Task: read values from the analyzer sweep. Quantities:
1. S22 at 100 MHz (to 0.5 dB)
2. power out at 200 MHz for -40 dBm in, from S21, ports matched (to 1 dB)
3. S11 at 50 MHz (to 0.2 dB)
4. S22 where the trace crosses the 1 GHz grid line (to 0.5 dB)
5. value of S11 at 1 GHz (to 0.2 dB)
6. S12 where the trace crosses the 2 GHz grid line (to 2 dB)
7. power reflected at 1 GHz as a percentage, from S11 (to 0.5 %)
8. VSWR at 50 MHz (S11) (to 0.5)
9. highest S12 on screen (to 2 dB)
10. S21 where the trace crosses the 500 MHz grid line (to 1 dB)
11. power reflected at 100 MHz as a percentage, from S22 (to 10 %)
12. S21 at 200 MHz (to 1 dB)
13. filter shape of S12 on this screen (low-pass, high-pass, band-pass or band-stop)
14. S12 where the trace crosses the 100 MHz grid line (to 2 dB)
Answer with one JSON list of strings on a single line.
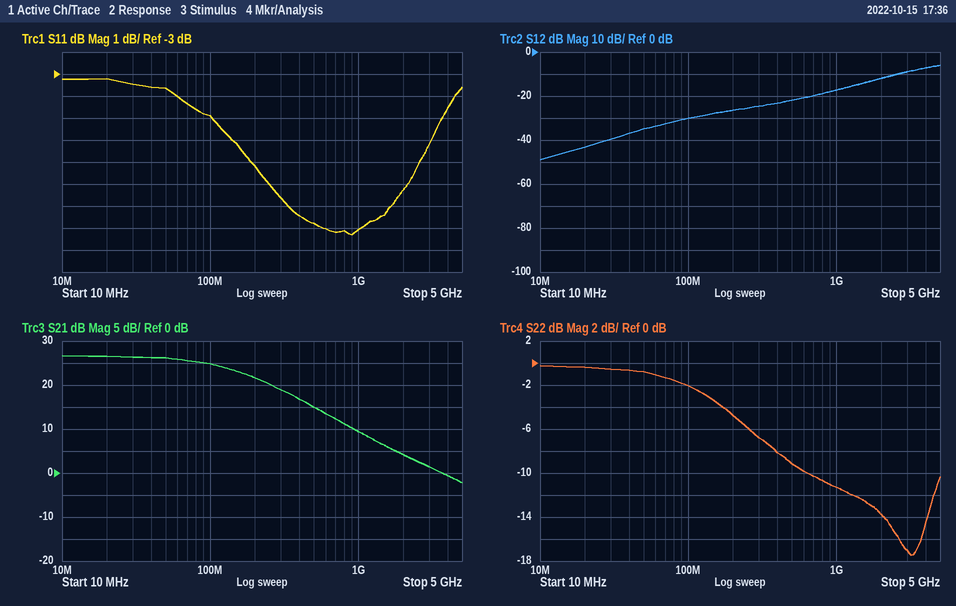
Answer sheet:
["-2.0 dB", "-18 dBm", "-3.6 dB", "-11.5 dB", "-10.0 dB", "-12 dB", "10.0 %", "5.0", "-6 dB", "15 dB", "60 %", "22 dB", "high-pass", "-30 dB"]
